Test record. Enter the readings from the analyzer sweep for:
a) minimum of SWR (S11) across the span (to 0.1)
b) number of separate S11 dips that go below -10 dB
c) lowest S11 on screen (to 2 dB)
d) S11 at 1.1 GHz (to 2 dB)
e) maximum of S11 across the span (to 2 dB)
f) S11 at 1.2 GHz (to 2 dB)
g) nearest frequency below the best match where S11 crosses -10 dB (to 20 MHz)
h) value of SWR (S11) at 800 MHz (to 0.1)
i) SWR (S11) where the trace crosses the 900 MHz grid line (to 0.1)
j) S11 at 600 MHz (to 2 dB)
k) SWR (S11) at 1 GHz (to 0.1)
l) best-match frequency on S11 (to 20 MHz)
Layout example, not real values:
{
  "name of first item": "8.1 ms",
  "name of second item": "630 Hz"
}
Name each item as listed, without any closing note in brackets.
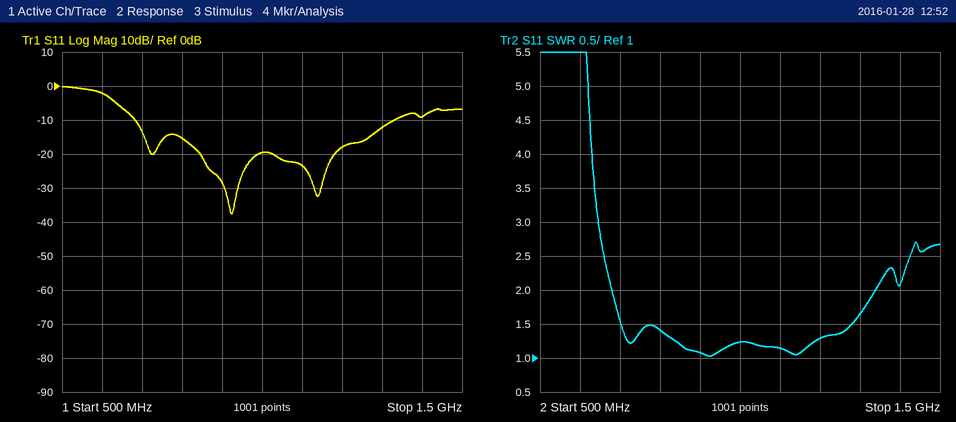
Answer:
{
  "minimum of SWR (S11) across the span": "1.0",
  "number of separate S11 dips that go below -10 dB": "3",
  "lowest S11 on screen": "-38 dB",
  "S11 at 1.1 GHz": "-24 dB",
  "maximum of S11 across the span": "0 dB",
  "S11 at 1.2 GHz": "-18 dB",
  "nearest frequency below the best match where S11 crosses -10 dB": "680 MHz",
  "value of SWR (S11) at 800 MHz": "1.4",
  "SWR (S11) where the trace crosses the 900 MHz grid line": "1.1",
  "S11 at 600 MHz": "-2 dB",
  "SWR (S11) at 1 GHz": "1.2",
  "best-match frequency on S11": "920 MHz"
}
